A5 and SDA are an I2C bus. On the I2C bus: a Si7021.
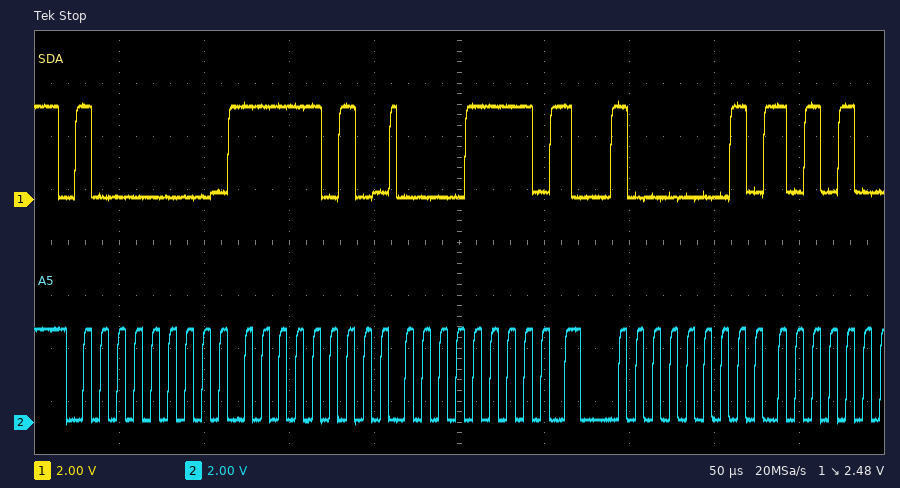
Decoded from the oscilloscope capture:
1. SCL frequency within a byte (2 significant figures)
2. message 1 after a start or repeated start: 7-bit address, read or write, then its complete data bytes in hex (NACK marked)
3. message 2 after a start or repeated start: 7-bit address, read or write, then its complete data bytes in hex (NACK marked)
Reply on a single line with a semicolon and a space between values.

100 kHz; 0x40 write: FA 0F; 0x40 read
